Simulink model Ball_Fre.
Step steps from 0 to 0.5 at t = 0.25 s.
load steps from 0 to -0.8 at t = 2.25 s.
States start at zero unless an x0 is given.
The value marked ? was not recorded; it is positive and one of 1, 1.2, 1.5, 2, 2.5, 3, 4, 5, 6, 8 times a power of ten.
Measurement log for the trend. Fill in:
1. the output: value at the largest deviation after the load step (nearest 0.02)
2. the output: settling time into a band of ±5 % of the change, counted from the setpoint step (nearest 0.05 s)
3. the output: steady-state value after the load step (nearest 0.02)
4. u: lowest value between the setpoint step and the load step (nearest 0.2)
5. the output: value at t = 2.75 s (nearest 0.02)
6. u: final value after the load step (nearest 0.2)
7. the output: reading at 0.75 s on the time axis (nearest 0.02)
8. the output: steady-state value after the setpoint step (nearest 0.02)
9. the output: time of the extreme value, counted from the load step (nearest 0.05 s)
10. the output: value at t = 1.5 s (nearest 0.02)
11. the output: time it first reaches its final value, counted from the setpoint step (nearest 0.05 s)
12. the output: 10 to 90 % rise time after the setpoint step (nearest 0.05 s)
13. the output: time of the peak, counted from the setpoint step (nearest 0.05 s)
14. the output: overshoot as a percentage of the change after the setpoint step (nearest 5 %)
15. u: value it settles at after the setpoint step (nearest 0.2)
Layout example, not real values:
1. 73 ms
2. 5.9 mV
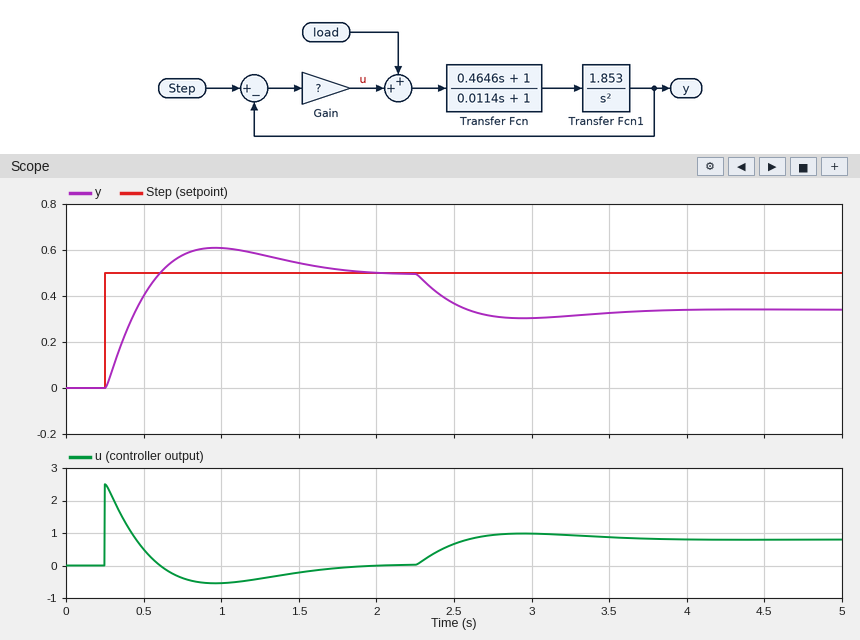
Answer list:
1. 0.30
2. 1.40 s
3. 0.34
4. -0.6
5. 0.32
6. 0.8
7. 0.58
8. 0.50
9. 0.70 s
10. 0.54
11. 0.35 s
12. 0.25 s
13. 0.70 s
14. 20 %
15. 0.0
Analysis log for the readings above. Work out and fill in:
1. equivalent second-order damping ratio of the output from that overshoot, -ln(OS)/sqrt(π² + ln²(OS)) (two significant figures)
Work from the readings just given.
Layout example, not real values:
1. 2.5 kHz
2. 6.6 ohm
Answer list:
1. 0.46
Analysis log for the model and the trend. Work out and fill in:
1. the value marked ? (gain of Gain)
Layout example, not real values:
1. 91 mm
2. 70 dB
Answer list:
1. 5
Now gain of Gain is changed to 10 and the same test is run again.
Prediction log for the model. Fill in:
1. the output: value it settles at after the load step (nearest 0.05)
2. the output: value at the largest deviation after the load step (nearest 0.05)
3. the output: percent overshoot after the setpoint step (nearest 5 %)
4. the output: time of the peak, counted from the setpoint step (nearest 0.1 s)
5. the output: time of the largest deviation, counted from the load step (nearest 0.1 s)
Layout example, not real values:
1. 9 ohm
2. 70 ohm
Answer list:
1. 0.40
2. 0.40
3. 15 %
4. 0.4 s
5. 0.4 s
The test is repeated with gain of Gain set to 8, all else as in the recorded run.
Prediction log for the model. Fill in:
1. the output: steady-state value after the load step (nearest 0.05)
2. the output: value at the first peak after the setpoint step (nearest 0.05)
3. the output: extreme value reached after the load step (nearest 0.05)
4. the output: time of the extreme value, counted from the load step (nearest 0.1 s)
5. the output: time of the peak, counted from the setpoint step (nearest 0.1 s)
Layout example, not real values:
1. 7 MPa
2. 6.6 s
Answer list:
1. 0.40
2. 0.60
3. 0.40
4. 0.5 s
5. 0.5 s
